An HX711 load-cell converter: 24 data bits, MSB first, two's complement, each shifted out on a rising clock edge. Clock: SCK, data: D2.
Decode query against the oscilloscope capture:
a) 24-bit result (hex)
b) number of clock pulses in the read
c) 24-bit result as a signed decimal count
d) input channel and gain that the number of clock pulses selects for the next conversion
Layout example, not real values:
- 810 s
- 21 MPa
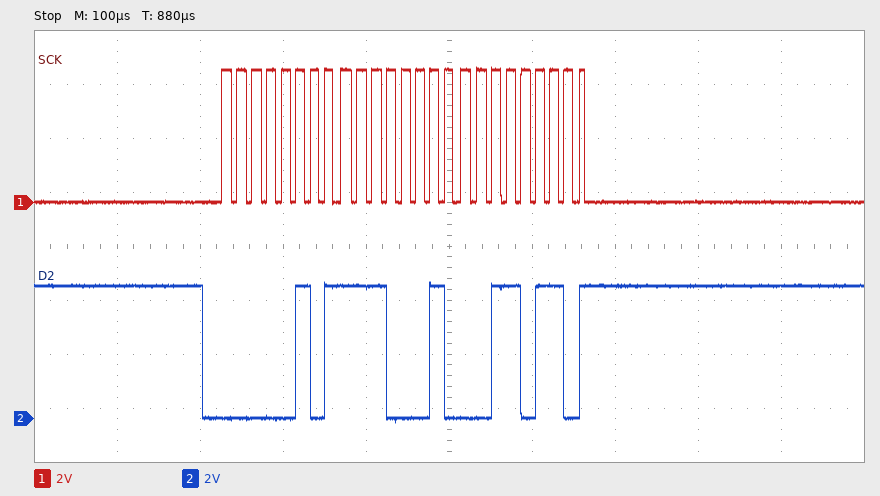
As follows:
- 0x05E236
- 25
- 385590
- channel A, gain 128
